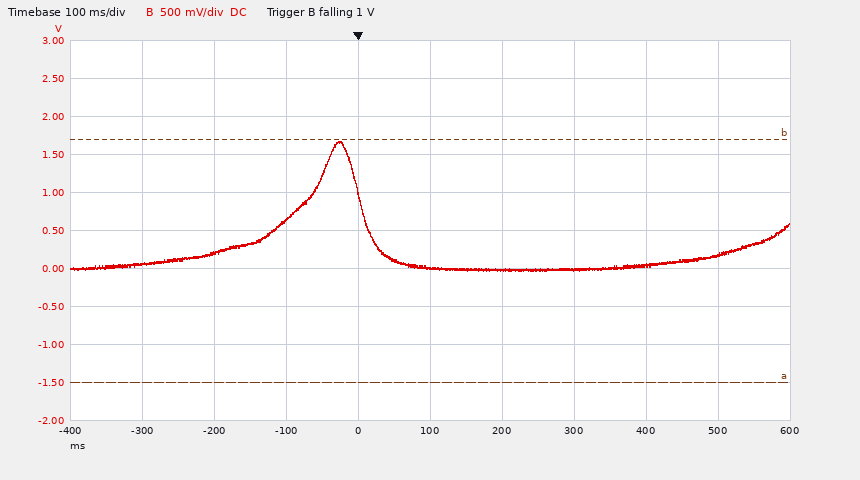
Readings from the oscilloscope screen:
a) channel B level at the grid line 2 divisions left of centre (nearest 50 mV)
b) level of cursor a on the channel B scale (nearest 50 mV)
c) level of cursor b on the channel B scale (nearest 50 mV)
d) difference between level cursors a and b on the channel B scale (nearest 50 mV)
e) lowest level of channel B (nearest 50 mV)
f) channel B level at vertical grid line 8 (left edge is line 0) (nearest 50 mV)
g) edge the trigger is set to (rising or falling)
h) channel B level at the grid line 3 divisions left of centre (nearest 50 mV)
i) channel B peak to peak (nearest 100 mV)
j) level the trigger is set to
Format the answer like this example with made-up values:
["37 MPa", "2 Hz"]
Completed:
["650 mV", "-1.50 V", "1.70 V", "3.20 V", "-50 mV", "50 mV", "falling", "200 mV", "1.70 V", "1 V"]
